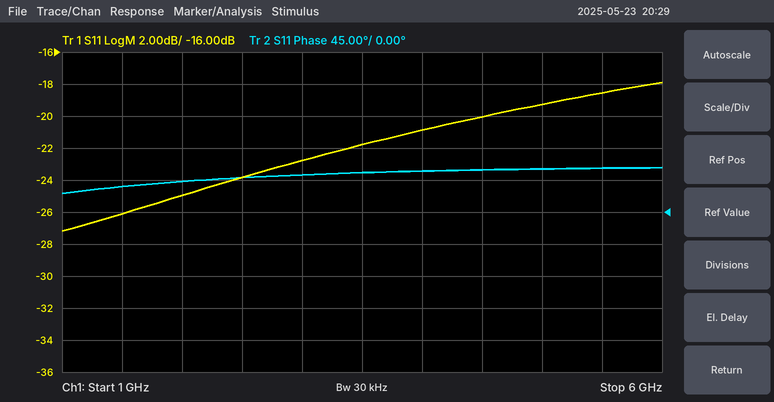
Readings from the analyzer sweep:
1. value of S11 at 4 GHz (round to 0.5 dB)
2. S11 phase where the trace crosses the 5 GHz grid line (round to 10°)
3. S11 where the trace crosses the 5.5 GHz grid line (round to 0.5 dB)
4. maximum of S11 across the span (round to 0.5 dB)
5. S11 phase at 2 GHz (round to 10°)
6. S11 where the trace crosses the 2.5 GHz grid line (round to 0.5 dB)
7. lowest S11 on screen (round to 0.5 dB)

-21.0 dB
60°
-18.5 dB
-18.0 dB
40°
-24.0 dB
-27.0 dB
